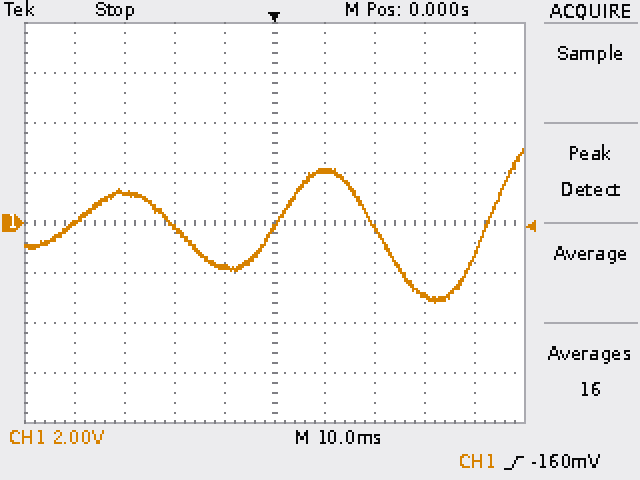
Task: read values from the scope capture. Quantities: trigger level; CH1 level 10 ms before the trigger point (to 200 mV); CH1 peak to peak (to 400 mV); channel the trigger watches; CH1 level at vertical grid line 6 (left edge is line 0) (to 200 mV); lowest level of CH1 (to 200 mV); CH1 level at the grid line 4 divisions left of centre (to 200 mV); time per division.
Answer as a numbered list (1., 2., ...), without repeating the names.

1. -160 mV
2. -1.8 V
3. 6.0 V
4. CH1
5. 2.0 V
6. -3.2 V
7. 0.0 V
8. 10 ms
